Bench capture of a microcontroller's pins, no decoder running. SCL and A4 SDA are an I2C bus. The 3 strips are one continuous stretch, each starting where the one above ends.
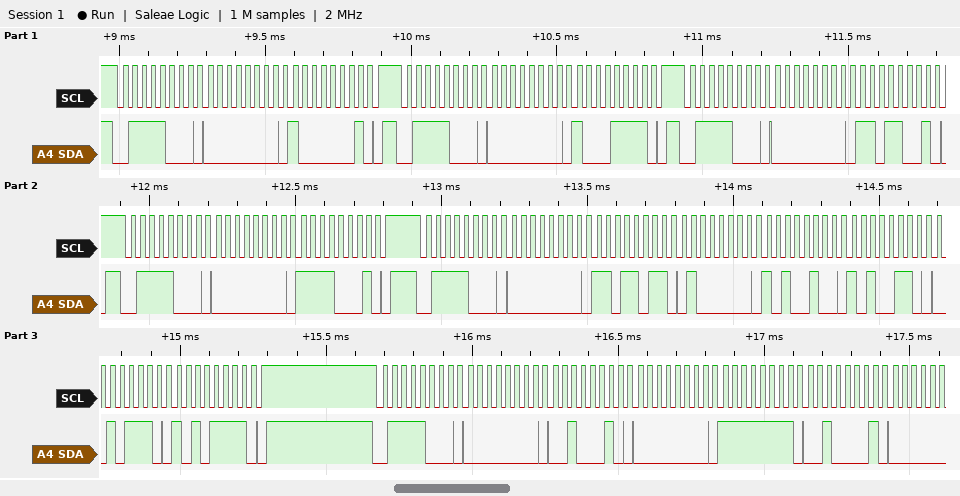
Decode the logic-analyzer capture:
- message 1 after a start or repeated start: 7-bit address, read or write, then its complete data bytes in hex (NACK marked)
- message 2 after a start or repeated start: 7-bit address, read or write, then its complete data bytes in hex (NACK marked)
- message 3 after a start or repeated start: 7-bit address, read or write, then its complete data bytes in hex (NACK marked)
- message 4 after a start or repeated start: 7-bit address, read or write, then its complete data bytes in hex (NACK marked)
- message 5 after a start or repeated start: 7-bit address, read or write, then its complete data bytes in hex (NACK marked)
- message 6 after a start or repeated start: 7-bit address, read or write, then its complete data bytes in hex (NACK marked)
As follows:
0x3C write: 00 81
0x3C write: 00 8F
0x3C write: 00 D9
0x3C write: 00 F1
0x3C write: 00 DB 40 A4 A6 2E AF
0x3C write: 00 22 00 FF 21
